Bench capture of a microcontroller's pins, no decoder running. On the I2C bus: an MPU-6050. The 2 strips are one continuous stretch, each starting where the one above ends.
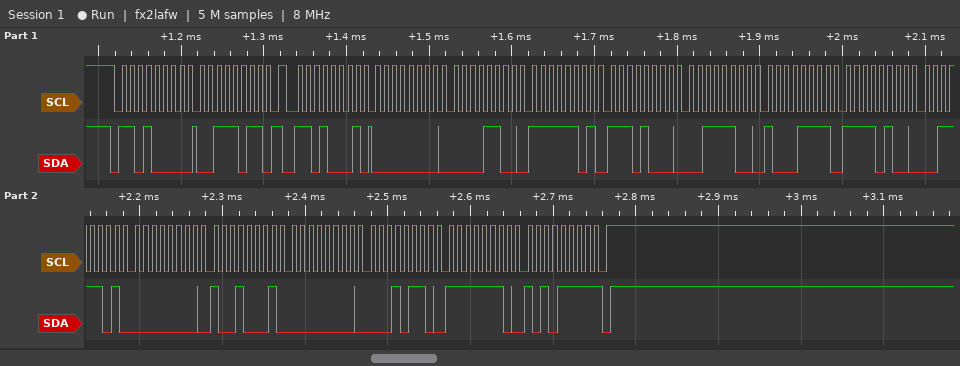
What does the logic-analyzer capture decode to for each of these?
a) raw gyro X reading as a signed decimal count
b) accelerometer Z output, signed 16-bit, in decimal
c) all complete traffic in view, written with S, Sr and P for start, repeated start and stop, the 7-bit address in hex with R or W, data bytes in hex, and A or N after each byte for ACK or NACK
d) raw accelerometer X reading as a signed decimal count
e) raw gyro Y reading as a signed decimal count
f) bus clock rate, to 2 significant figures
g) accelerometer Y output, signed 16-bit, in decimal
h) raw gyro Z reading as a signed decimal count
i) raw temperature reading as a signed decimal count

145
15503
S 68W A 3B A Sr 68R A 00 A 0C A FD A E8 A 3C A 8F A F4 A 3D A 00 A 91 A 00 A 16 A FE A AF N P
12
22
100 kHz
-536
-337
-3011
